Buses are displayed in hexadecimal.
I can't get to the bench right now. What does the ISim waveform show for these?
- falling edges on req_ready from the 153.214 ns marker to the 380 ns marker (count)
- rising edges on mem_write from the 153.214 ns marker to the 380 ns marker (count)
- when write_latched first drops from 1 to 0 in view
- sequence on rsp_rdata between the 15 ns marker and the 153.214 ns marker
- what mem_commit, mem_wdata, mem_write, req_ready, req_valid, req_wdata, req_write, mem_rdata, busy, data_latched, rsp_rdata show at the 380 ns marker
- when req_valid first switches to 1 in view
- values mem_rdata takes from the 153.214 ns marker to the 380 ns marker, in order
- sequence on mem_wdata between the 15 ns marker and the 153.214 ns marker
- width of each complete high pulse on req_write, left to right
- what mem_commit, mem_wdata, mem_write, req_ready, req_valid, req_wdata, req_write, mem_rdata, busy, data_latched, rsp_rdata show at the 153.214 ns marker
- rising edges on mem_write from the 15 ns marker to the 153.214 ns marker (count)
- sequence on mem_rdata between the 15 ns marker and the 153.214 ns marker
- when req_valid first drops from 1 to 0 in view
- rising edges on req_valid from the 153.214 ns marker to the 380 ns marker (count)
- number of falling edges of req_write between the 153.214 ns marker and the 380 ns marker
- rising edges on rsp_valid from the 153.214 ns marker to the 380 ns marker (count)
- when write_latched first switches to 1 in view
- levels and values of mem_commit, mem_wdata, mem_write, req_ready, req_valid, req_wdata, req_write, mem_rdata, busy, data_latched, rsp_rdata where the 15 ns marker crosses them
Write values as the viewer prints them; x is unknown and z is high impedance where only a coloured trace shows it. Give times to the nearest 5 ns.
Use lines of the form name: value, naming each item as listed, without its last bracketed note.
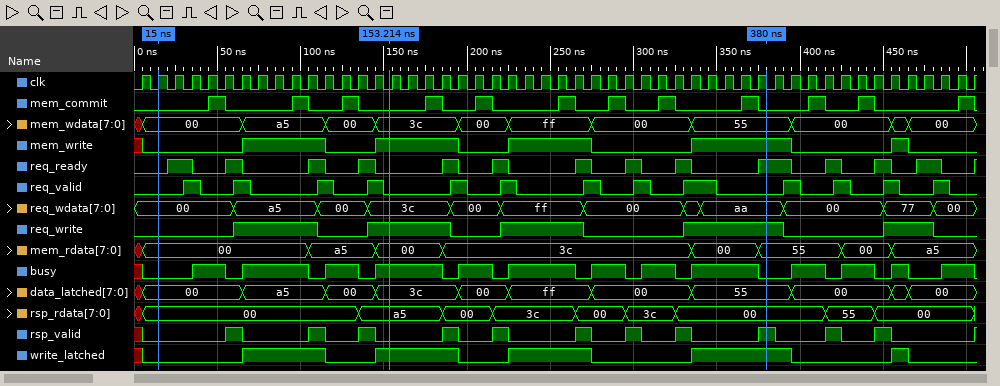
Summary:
falling edges on req_ready from the 153.214 ns marker to the 380 ns marker: 5
rising edges on mem_write from the 153.214 ns marker to the 380 ns marker: 2
when write_latched first drops from 1 to 0 in view: 115 ns
sequence on rsp_rdata between the 15 ns marker and the 153.214 ns marker: 00, a5
what mem_commit, mem_wdata, mem_write, req_ready, req_valid, req_wdata, req_write, mem_rdata, busy, data_latched, rsp_rdata show at the 380 ns marker: mem_commit=0, mem_wdata=55, mem_write=1, req_ready=1, req_valid=0, req_wdata=aa, req_write=1, mem_rdata=55, busy=0, data_latched=55, rsp_rdata=00
when req_valid first switches to 1 in view: 30 ns
values mem_rdata takes from the 153.214 ns marker to the 380 ns marker, in order: 00, 3c, 00, 55
sequence on mem_wdata between the 15 ns marker and the 153.214 ns marker: 00, a5, 00, 3c
width of each complete high pulse on req_write, left to right: 50 ns, 50 ns, 50 ns, 60 ns, 30 ns
what mem_commit, mem_wdata, mem_write, req_ready, req_valid, req_wdata, req_write, mem_rdata, busy, data_latched, rsp_rdata show at the 153.214 ns marker: mem_commit=0, mem_wdata=3c, mem_write=1, req_ready=0, req_valid=0, req_wdata=3c, req_write=1, mem_rdata=00, busy=1, data_latched=3c, rsp_rdata=a5
rising edges on mem_write from the 15 ns marker to the 153.214 ns marker: 2
sequence on mem_rdata between the 15 ns marker and the 153.214 ns marker: 00, a5, 00
when req_valid first drops from 1 to 0 in view: 40 ns
rising edges on req_valid from the 153.214 ns marker to the 380 ns marker: 5
number of falling edges of req_write between the 153.214 ns marker and the 380 ns marker: 2
rising edges on rsp_valid from the 153.214 ns marker to the 380 ns marker: 6
when write_latched first switches to 1 in view: 65 ns
levels and values of mem_commit, mem_wdata, mem_write, req_ready, req_valid, req_wdata, req_write, mem_rdata, busy, data_latched, rsp_rdata where the 15 ns marker crosses them: mem_commit=0, mem_wdata=00, mem_write=0, req_ready=0, req_valid=0, req_wdata=00, req_write=0, mem_rdata=00, busy=0, data_latched=00, rsp_rdata=00
